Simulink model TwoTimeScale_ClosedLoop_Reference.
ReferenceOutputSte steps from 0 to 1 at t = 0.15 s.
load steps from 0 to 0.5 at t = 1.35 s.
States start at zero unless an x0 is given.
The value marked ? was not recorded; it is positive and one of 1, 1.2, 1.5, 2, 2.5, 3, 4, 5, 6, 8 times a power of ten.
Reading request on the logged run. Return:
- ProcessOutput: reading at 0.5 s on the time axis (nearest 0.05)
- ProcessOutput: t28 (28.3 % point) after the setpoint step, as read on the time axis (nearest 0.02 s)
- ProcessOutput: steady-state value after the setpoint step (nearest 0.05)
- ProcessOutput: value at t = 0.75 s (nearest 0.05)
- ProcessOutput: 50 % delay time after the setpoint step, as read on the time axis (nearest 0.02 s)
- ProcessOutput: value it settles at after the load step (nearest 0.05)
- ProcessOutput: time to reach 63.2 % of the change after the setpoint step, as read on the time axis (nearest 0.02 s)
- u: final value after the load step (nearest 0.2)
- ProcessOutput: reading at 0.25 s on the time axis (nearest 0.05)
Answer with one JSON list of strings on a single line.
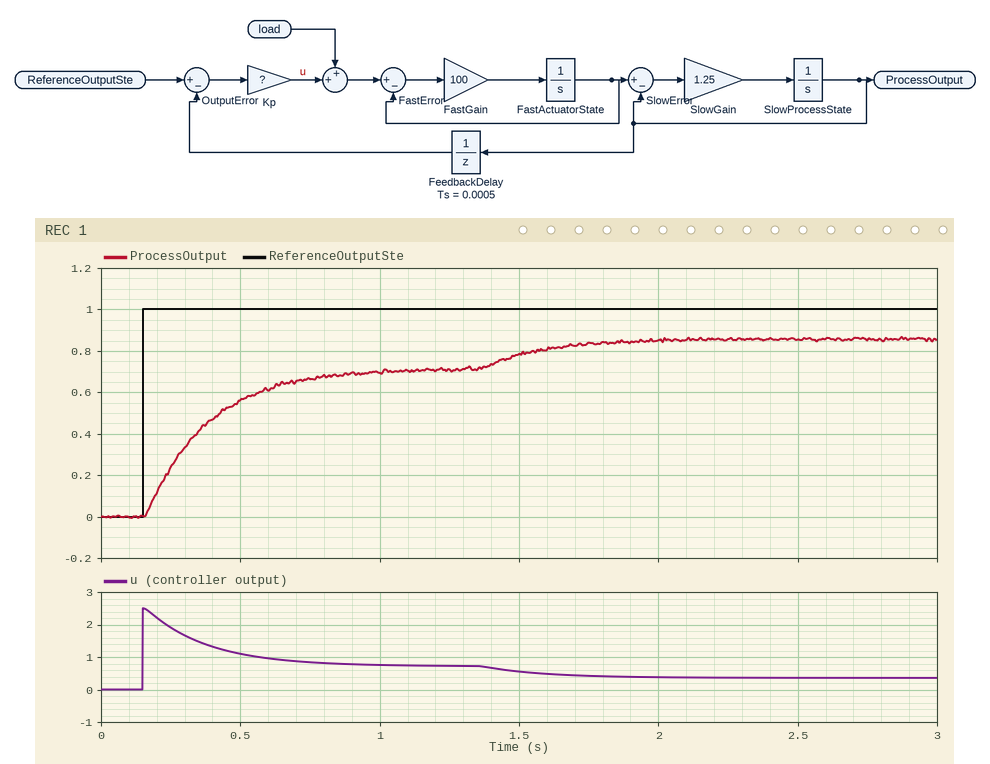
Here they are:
["0.55", "0.24 s", "0.70", "0.65", "0.32 s", "0.85", "0.38 s", "0.4", "0.25"]
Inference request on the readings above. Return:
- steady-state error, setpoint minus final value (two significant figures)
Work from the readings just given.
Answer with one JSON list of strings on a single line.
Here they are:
["0.30"]
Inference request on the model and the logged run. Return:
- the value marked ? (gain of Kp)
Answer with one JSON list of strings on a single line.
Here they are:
["2.5"]
